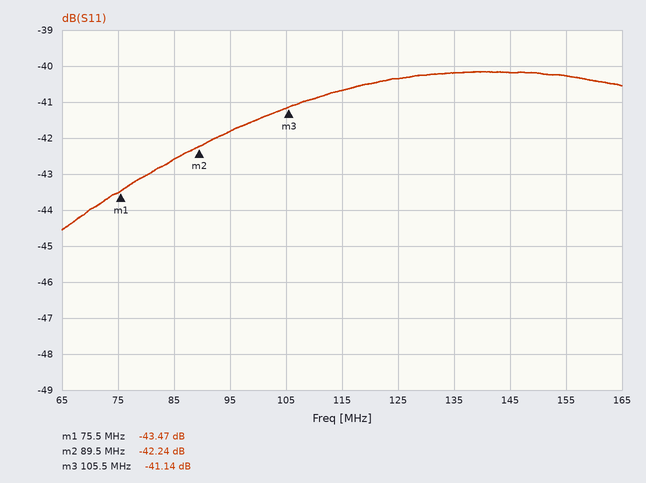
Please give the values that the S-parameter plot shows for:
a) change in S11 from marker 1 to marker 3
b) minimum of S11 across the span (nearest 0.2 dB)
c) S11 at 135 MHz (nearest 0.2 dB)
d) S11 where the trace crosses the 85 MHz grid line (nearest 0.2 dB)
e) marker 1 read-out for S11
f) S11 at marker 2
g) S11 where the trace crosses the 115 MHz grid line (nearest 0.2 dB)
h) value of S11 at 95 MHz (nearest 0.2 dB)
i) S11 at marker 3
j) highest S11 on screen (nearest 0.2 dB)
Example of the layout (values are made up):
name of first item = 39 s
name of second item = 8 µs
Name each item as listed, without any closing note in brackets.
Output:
change in S11 from marker 1 to marker 3 = 2.33 dB
minimum of S11 across the span = -44.6 dB
S11 at 135 MHz = -40.2 dB
S11 where the trace crosses the 85 MHz grid line = -42.6 dB
marker 1 read-out for S11 = -43.47 dB
S11 at marker 2 = -42.24 dB
S11 where the trace crosses the 115 MHz grid line = -40.6 dB
value of S11 at 95 MHz = -41.8 dB
S11 at marker 3 = -41.14 dB
highest S11 on screen = -40.2 dB
